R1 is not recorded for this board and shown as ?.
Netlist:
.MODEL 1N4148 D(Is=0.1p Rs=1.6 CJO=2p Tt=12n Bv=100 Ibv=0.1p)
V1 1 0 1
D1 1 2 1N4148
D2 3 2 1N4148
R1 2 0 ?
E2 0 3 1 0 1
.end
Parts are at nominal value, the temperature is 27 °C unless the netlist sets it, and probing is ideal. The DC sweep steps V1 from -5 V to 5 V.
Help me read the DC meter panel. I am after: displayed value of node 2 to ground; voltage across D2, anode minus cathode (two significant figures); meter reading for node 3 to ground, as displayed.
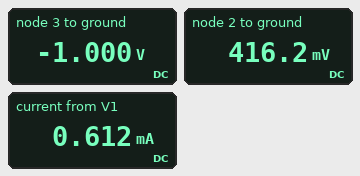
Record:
416.2 mV
-1.4 V
-1.000 V
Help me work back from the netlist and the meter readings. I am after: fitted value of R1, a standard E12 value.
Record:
680 Ω
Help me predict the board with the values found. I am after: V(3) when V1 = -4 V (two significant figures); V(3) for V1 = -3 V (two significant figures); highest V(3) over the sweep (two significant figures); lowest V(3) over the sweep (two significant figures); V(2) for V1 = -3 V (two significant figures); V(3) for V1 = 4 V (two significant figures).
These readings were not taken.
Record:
4.0 V
3.0 V
5.0 V
-5.0 V
2.4 V
-4.0 V
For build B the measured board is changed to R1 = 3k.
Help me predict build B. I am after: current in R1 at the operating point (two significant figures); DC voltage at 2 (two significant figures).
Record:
150 µA
450 mV
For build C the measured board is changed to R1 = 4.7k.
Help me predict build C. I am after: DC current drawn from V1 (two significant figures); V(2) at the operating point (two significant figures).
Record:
99 µA
460 mV
